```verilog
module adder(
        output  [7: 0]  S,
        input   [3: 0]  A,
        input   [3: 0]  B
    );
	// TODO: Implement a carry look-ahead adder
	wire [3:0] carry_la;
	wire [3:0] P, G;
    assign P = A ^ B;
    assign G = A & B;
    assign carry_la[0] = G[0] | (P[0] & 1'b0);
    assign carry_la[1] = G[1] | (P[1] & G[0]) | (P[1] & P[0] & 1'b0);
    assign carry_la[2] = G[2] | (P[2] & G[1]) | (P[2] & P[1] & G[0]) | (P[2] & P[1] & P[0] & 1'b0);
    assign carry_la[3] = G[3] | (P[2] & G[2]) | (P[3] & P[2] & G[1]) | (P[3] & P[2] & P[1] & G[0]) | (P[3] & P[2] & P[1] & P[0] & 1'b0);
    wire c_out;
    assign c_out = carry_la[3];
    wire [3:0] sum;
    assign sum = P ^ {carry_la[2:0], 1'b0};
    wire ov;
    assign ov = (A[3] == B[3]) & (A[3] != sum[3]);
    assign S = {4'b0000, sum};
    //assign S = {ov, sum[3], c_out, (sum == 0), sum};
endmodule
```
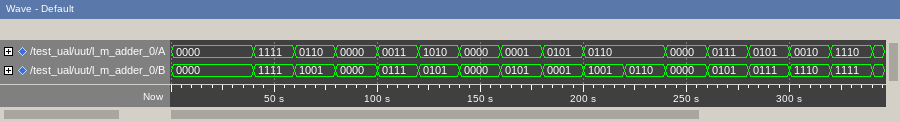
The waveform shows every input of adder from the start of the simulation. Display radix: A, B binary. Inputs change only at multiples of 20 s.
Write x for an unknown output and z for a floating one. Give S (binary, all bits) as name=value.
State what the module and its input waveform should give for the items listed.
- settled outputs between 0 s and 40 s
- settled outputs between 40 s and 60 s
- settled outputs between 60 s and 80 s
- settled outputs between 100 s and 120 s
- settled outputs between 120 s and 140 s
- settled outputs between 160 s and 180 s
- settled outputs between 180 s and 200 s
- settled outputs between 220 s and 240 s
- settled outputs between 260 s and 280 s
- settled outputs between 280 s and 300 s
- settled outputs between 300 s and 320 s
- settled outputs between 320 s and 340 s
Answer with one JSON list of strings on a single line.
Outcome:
["S=00000000", "S=00001110", "S=00001111", "S=00001010", "S=00001111", "S=00000110", "S=00000110", "S=00001100", "S=00001100", "S=00001100", "S=00000000", "S=00001101"]
